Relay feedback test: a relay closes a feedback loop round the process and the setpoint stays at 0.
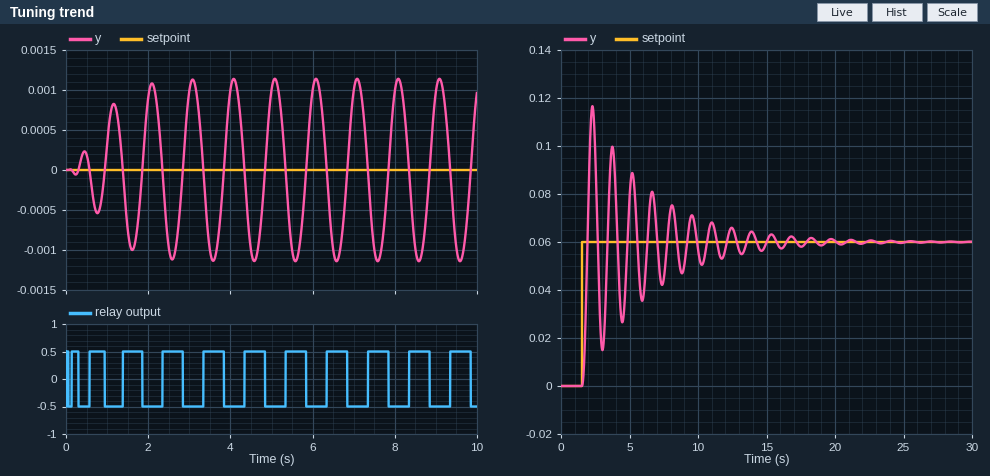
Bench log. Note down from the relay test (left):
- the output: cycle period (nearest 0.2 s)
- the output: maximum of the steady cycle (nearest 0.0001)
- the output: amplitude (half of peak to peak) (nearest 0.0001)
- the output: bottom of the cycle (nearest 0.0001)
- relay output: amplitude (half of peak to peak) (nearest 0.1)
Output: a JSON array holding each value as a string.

["1.0 s", "0.0011", "0.0011", "-0.0011", "0.5"]
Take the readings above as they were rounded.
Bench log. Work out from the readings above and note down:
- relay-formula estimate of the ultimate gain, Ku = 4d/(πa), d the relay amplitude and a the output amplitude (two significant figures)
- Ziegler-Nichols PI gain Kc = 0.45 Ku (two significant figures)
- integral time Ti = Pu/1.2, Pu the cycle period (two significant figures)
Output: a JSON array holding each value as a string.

["580", "260", "0.83 s"]
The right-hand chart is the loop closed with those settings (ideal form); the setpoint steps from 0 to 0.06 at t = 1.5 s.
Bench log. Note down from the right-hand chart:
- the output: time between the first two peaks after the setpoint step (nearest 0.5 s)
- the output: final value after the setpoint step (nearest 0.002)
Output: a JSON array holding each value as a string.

["1.5 s", "0.060"]
